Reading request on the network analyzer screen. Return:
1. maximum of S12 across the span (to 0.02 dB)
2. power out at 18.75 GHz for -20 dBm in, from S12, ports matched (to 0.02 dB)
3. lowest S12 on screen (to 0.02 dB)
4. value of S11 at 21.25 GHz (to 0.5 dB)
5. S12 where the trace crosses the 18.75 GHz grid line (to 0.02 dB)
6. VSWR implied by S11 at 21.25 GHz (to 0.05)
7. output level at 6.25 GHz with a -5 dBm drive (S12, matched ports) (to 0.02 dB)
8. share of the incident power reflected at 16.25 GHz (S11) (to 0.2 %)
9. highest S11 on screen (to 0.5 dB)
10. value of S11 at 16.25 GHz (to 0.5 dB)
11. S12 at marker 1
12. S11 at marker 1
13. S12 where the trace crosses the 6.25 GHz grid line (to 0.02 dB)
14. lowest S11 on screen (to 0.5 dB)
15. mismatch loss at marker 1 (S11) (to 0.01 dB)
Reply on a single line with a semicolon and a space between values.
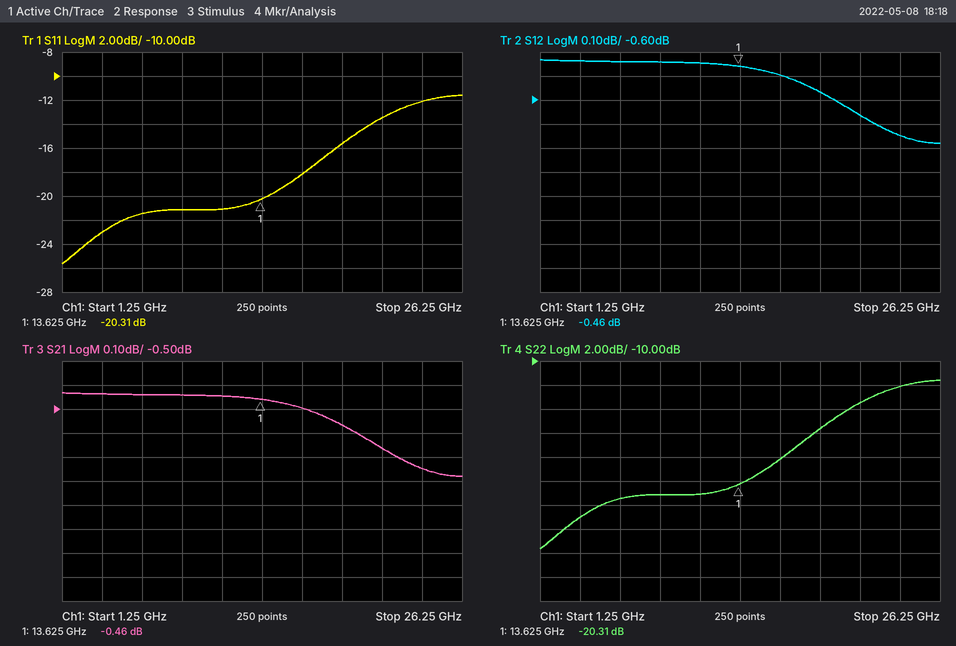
-0.44 dB; -20.56 dBm; -0.78 dB; -13.5 dB; -0.56 dB; 1.55; -5.44 dBm; 1.6 %; -11.5 dB; -18.0 dB; -0.46 dB; -20.31 dB; -0.44 dB; -25.5 dB; 0.04 dB
